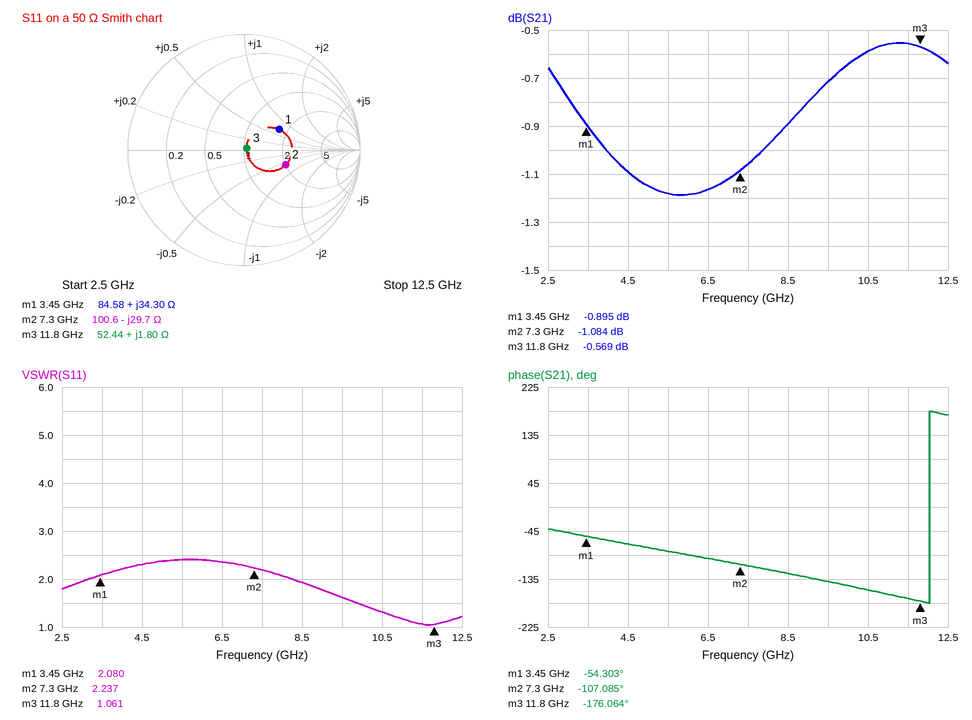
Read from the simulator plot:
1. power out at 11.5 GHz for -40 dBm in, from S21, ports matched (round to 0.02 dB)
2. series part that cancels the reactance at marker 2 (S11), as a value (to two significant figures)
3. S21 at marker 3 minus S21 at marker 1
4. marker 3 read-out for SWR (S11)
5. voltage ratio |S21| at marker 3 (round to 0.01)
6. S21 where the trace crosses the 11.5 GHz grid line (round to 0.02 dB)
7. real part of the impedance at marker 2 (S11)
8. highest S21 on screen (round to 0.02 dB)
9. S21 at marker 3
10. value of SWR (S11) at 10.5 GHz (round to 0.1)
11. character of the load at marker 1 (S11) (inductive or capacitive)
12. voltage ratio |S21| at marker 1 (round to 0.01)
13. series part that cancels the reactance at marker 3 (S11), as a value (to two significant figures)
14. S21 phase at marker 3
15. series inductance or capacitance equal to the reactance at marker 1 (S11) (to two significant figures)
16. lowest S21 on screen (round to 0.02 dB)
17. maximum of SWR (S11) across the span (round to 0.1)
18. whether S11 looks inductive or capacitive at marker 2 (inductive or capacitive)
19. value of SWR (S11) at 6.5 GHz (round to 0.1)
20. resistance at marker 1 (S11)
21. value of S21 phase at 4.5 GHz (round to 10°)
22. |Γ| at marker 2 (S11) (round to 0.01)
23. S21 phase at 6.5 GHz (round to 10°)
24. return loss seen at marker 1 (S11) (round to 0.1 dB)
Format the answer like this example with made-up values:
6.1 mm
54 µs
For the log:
-40.56 dBm
650 pH
0.326 dB
1.061
0.94
-0.56 dB
100.6 Ω
-0.56 dB
-0.569 dB
1.3
inductive
0.90
7.5 pF
-176.064°
1.6 nH
-1.18 dB
2.4
capacitive
2.4
84.58 Ω
-70°
0.38
-100°
9.1 dB
